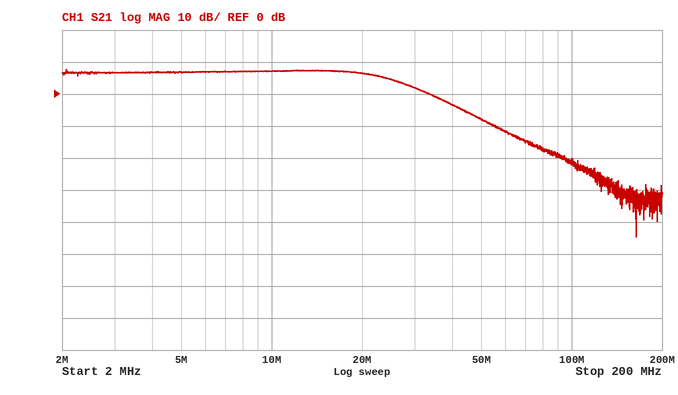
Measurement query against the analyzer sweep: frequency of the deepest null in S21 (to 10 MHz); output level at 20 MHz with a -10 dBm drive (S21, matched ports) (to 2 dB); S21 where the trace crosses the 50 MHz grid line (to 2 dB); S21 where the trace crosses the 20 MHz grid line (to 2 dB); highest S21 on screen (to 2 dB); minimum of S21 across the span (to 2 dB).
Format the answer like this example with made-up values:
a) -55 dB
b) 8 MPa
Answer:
a) 160 MHz
b) -4 dBm
c) -8 dB
d) 6 dB
e) 8 dB
f) -44 dB
